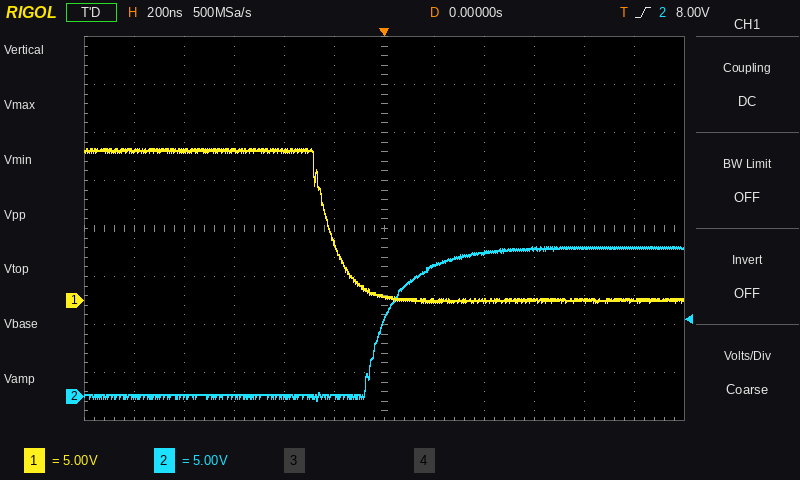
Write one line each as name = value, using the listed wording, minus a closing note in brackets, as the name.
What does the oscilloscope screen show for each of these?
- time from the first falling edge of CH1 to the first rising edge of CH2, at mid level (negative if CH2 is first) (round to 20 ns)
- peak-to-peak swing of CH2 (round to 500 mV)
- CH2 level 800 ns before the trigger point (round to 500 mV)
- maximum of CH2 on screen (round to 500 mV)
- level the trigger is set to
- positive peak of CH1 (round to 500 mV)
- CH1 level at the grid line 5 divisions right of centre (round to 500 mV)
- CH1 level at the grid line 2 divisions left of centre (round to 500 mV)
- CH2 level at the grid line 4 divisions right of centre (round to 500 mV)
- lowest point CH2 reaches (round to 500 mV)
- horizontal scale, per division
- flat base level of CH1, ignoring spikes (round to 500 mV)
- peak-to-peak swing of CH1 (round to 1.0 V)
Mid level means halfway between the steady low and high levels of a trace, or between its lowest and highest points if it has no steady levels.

time from the first falling edge of CH1 to the first rising edge of CH2, at mid level (negative if CH2 is first) = +220 ns
peak-to-peak swing of CH2 = 16.0 V
CH2 level 800 ns before the trigger point = 0.0 V
maximum of CH2 on screen = 15.5 V
level the trigger is set to = 8.00 V
positive peak of CH1 = 16.0 V
CH1 level at the grid line 5 divisions right of centre = 0.0 V
CH1 level at the grid line 2 divisions left of centre = 15.5 V
CH2 level at the grid line 4 divisions right of centre = 15.5 V
lowest point CH2 reaches = -500 mV
horizontal scale, per division = 200 ns
flat base level of CH1, ignoring spikes = 0.0 V
peak-to-peak swing of CH1 = 16.0 V
